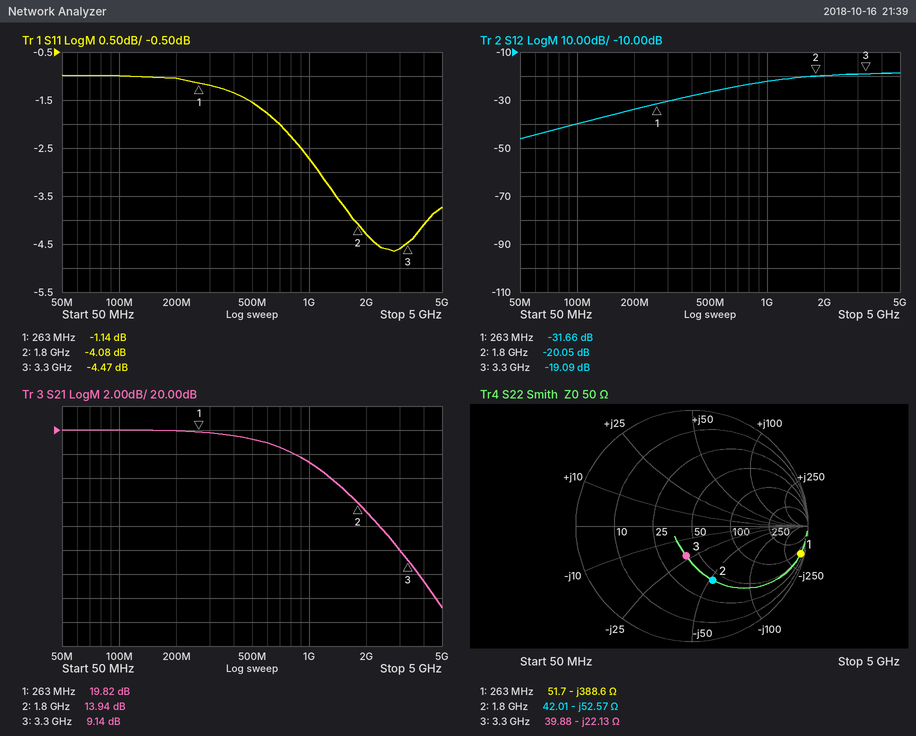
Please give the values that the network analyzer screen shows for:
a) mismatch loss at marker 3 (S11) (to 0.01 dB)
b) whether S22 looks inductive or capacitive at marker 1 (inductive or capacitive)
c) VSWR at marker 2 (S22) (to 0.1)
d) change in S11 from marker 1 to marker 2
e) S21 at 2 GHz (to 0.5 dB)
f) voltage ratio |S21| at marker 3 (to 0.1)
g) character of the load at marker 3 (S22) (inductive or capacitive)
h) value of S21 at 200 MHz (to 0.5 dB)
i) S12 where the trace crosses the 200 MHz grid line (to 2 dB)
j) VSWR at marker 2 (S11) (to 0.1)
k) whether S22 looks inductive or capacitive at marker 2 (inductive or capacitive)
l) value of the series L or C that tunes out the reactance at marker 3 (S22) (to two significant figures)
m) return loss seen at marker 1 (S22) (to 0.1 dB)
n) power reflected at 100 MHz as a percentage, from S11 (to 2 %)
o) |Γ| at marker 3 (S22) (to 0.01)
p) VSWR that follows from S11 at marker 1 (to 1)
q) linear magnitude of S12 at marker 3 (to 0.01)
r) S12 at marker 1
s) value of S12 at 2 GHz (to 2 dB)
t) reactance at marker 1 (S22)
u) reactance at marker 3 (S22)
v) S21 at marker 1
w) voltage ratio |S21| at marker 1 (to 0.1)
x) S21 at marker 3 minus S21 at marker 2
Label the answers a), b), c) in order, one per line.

a) 1.92 dB
b) capacitive
c) 3.0
d) -2.94 dB
e) 13.0 dB
f) 2.9
g) capacitive
h) 20.0 dB
i) -34 dB
j) 4.3
k) capacitive
l) 1.1 nH
m) 0.3 dB
n) 80 %
o) 0.26
p) 15
q) 0.11
r) -31.66 dB
s) -20 dB
t) -388.6 Ω
u) -22.13 Ω
v) 19.82 dB
w) 9.8
x) -4.80 dB
